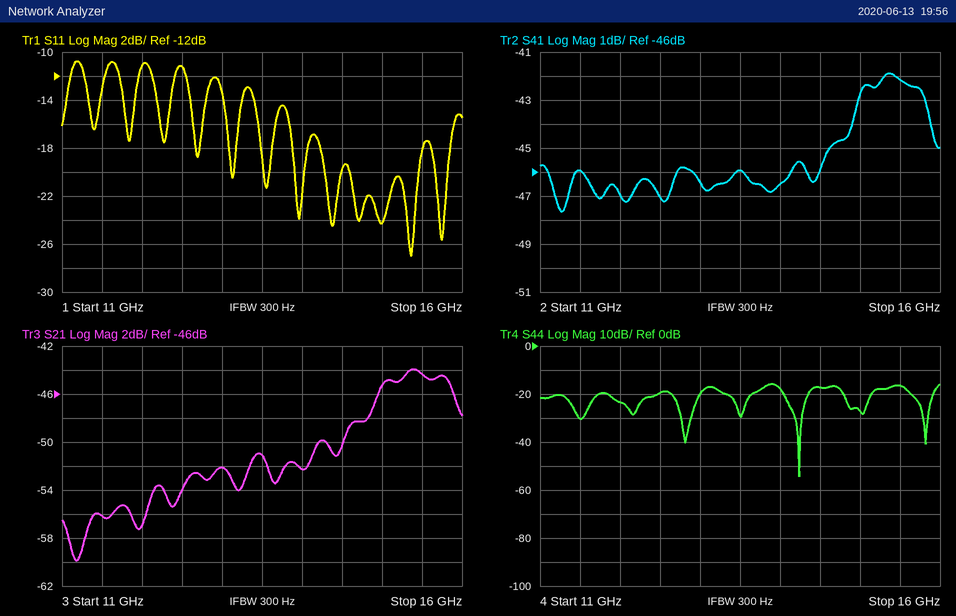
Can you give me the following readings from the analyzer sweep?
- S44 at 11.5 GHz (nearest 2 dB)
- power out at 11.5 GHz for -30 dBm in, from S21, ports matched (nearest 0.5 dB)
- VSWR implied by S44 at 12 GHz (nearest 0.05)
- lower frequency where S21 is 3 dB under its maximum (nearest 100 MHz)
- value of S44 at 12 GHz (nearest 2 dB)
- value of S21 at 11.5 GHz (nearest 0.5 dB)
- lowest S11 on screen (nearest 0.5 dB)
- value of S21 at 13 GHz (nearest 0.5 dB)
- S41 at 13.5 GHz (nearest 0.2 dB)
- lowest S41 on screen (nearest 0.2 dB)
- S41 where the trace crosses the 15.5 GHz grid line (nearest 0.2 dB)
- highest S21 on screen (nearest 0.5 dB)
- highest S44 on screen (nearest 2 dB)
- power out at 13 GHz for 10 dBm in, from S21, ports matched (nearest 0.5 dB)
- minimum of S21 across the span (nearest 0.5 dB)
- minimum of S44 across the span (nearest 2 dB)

-30 dB
-86.0 dBm
1.15
14.9 GHz
-24 dB
-56.0 dB
-27.0 dB
-52.0 dB
-46.0 dB
-47.6 dB
-42.2 dB
-44.0 dB
-16 dB
-42.0 dBm
-60.0 dB
-54 dB
